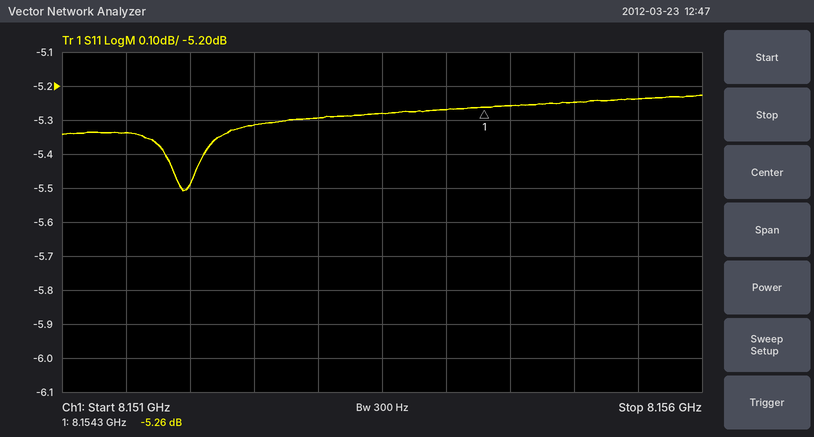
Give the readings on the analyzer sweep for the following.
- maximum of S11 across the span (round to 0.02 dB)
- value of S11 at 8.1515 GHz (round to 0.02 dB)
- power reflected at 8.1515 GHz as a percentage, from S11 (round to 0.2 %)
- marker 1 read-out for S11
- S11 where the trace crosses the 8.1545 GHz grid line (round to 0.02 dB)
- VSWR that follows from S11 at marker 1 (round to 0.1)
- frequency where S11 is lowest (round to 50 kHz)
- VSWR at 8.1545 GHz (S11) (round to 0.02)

-5.22 dB
-5.34 dB
29.2 %
-5.26 dB
-5.26 dB
3.4
8.15195 GHz
3.40
